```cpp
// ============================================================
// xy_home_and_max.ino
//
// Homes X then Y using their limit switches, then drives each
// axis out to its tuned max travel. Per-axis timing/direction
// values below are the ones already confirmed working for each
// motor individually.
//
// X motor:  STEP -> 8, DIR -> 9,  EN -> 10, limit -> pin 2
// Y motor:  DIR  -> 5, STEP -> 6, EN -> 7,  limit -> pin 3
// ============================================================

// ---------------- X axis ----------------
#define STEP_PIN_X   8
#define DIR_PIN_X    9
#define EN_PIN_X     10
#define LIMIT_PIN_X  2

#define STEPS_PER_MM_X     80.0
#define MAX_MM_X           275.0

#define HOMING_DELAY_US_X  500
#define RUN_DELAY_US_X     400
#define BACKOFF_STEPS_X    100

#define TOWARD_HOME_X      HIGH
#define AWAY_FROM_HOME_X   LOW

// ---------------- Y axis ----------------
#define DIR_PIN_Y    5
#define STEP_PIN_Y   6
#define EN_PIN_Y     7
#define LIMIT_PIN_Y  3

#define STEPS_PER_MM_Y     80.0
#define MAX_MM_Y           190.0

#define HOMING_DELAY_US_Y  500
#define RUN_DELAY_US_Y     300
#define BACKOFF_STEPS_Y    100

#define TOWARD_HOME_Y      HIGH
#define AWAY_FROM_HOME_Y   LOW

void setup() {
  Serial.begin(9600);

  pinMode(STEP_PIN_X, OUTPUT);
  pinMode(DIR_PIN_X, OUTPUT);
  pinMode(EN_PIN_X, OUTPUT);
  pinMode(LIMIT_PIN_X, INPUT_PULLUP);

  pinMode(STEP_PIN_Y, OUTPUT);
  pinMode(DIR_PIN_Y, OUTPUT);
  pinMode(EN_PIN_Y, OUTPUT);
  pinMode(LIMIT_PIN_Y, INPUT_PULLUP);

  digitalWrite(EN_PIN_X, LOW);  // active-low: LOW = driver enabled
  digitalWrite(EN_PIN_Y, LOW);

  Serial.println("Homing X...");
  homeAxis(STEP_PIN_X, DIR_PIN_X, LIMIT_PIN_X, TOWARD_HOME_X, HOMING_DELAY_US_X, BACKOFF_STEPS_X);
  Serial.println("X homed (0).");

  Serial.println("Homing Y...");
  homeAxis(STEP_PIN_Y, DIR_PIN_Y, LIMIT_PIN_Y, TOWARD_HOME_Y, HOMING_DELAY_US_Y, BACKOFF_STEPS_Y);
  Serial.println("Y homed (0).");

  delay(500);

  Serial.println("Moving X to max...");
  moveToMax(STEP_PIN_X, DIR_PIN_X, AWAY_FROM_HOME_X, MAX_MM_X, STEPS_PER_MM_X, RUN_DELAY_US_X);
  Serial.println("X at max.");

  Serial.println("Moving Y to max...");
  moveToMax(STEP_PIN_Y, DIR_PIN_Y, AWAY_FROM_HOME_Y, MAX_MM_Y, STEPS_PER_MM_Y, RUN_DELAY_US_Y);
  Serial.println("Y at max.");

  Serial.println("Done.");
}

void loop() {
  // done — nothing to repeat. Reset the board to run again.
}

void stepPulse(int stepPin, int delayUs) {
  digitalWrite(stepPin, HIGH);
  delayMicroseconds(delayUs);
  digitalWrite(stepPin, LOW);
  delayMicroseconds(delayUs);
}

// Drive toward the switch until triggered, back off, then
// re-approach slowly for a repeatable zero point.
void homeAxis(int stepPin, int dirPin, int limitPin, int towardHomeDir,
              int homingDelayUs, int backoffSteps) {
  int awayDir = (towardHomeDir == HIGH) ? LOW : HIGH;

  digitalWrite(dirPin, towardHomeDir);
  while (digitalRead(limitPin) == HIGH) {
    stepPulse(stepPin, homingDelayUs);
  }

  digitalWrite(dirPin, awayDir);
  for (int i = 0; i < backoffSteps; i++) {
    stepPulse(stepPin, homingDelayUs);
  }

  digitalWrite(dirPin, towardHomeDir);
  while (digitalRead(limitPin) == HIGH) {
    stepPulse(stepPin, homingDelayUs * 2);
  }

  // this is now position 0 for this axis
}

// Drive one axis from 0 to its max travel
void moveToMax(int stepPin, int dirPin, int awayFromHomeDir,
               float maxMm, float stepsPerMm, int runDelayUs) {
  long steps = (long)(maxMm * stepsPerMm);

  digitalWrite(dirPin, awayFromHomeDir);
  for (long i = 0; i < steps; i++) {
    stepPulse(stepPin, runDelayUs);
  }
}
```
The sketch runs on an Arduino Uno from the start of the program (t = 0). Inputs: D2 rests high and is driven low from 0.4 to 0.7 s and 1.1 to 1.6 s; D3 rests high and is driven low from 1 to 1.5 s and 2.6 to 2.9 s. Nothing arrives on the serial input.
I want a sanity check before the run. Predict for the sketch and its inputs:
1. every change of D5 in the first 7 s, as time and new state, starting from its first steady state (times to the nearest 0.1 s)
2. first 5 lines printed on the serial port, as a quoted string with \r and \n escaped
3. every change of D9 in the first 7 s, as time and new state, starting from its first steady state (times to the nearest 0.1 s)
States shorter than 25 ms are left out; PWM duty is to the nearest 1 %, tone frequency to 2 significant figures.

0 s low; 0.5 s high; 1 s low; 1.1 s high
"Homing X...\r\nX homed (0).\r\nHoming Y...\r\nY homed (0).\r\nMoving X to max...\r\n"
0 s high; 0.4 s low; 0.5 s high; 1.6 s low
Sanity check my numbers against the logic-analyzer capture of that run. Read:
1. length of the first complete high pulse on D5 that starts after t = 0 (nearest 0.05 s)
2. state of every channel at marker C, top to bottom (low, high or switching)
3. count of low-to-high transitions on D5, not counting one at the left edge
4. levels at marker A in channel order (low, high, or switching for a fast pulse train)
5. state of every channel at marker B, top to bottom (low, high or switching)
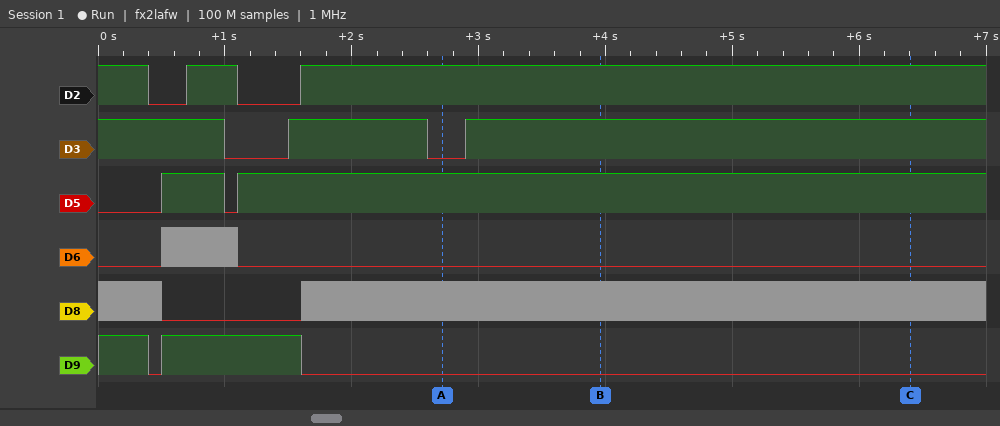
0.50 s
D2 high, D3 high, D5 high, D6 low, D8 switching, D9 low
2
D2 high, D3 low, D5 high, D6 low, D8 switching, D9 low
D2 high, D3 high, D5 high, D6 low, D8 switching, D9 low
